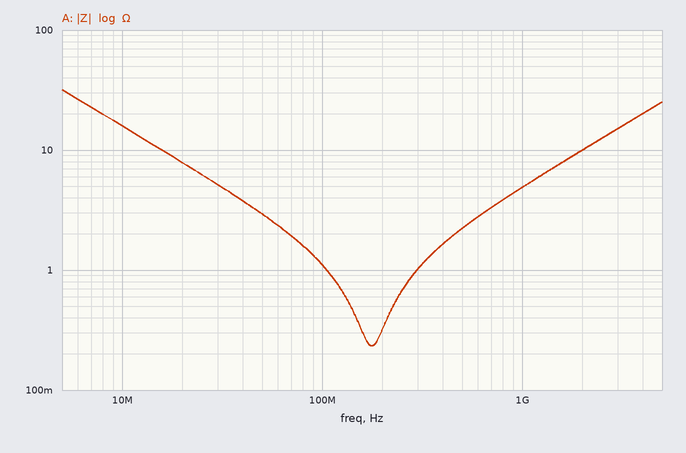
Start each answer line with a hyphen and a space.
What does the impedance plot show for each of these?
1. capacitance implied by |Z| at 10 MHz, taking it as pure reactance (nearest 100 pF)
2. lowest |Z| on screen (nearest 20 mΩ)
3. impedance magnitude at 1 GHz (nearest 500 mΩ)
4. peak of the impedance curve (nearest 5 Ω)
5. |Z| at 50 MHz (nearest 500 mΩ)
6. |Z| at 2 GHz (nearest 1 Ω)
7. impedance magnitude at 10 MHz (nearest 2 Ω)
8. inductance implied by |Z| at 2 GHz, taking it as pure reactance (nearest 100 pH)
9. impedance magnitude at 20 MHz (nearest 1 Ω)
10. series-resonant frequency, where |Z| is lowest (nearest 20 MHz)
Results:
- 1.0 nF
- 240 mΩ
- 5.0 Ω
- 30 Ω
- 3.0 Ω
- 10 Ω
- 16 Ω
- 800 pH
- 8 Ω
- 180 MHz
